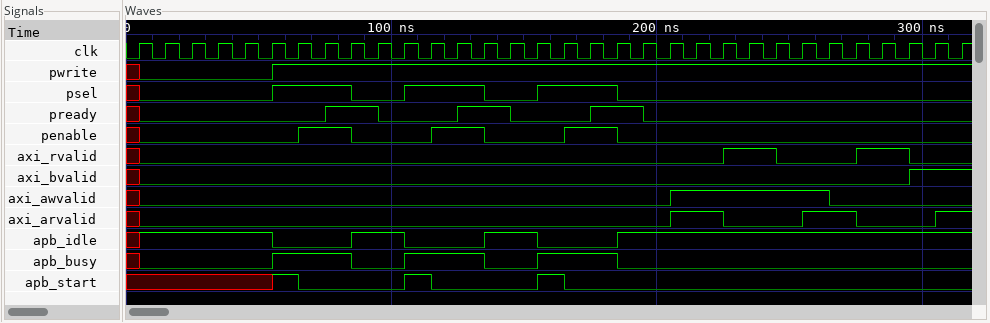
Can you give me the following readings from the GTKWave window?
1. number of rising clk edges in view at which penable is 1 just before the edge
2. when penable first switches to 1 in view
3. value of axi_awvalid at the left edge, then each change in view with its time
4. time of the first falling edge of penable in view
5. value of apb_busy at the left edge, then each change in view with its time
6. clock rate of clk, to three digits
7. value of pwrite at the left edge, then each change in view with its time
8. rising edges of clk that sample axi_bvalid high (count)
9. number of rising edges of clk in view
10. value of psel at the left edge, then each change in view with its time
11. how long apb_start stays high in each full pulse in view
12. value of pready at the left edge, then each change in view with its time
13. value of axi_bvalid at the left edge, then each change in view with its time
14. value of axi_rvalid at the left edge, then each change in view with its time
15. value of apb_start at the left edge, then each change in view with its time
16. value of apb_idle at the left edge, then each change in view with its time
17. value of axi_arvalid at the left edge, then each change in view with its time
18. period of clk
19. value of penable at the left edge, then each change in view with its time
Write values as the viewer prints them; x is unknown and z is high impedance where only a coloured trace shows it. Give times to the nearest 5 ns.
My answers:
6
65 ns
x, 0 at 5 ns, 1 at 205 ns, 0 at 265 ns
85 ns
x, 0 at 5 ns, 1 at 55 ns, 0 at 85 ns, 1 at 105 ns, 0 at 135 ns, 1 at 155 ns, 0 at 185 ns
100 MHz
x, 0 at 5 ns, 1 at 55 ns
2
32
x, 0 at 5 ns, 1 at 55 ns, 0 at 85 ns, 1 at 105 ns, 0 at 135 ns, 1 at 155 ns, 0 at 185 ns
10 ns, 10 ns
x, 0 at 5 ns, 1 at 75 ns, 0 at 95 ns, 1 at 125 ns, 0 at 145 ns, 1 at 175 ns, 0 at 195 ns
x, 0 at 5 ns, 1 at 295 ns
x, 0 at 5 ns, 1 at 225 ns, 0 at 245 ns, 1 at 275 ns, 0 at 295 ns
x, 1 at 55 ns, 0 at 65 ns, 1 at 105 ns, 0 at 115 ns, 1 at 155 ns, 0 at 165 ns
x, 1 at 5 ns, 0 at 55 ns, 1 at 85 ns, 0 at 105 ns, 1 at 135 ns, 0 at 155 ns, 1 at 185 ns
x, 0 at 5 ns, 1 at 205 ns, 0 at 225 ns, 1 at 255 ns, 0 at 275 ns, 1 at 305 ns
10 ns
x, 0 at 5 ns, 1 at 65 ns, 0 at 85 ns, 1 at 115 ns, 0 at 135 ns, 1 at 165 ns, 0 at 185 ns
